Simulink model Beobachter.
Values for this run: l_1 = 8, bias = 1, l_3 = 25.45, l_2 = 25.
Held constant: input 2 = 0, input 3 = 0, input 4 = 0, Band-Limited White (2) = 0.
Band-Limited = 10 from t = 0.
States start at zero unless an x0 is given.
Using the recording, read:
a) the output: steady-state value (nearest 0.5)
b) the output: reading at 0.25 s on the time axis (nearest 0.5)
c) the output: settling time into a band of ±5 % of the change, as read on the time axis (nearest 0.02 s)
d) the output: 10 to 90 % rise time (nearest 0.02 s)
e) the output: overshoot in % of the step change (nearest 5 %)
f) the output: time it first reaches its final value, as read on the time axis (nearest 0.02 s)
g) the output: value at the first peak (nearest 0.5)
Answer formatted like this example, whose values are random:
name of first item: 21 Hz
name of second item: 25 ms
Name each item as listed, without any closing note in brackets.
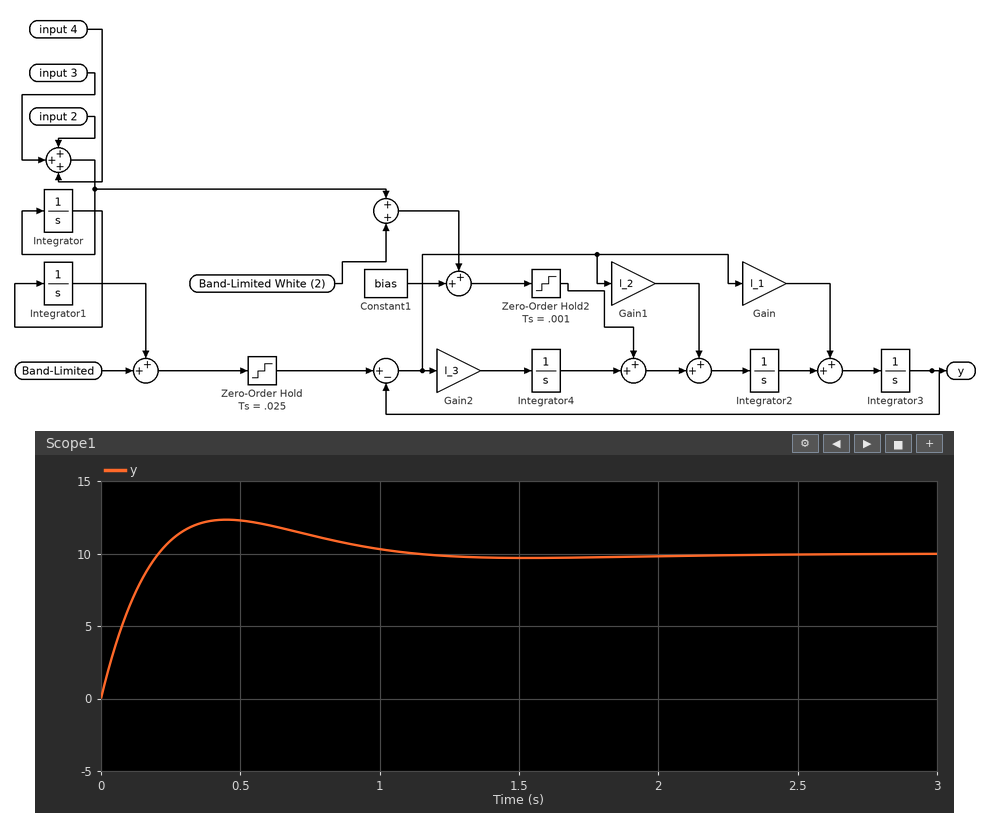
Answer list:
the output: steady-state value: 10.0
the output: reading at 0.25 s on the time axis: 11.0
the output: settling time into a band of ±5 % of the change, as read on the time axis: 0.94 s
the output: 10 to 90 % rise time: 0.16 s
the output: overshoot in % of the step change: 25 %
the output: time it first reaches its final value, as read on the time axis: 0.20 s
the output: value at the first peak: 12.5
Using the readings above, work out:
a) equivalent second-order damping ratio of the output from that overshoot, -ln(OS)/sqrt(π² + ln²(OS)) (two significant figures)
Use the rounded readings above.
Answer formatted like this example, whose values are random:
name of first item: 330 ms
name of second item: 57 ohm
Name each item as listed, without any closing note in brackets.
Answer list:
equivalent second-order damping ratio of the output from that overshoot, -ln(OS)/sqrt(π² + ln²(OS)): 0.40
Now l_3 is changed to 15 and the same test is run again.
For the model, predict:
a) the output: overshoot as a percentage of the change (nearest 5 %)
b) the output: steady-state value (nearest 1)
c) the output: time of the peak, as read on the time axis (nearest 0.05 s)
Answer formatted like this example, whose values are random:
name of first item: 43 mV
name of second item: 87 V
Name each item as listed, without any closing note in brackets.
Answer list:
the output: overshoot as a percentage of the change: 20 %
the output: steady-state value: 10
the output: time of the peak, as read on the time axis: 0.45 s
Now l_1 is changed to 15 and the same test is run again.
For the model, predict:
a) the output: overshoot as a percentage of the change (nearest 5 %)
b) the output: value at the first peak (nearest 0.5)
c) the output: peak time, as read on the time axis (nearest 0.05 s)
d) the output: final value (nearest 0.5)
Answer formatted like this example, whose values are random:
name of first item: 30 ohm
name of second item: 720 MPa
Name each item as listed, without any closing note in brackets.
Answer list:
the output: overshoot as a percentage of the change: 10 %
the output: value at the first peak: 11.0
the output: peak time, as read on the time axis: 0.40 s
the output: final value: 10.0
